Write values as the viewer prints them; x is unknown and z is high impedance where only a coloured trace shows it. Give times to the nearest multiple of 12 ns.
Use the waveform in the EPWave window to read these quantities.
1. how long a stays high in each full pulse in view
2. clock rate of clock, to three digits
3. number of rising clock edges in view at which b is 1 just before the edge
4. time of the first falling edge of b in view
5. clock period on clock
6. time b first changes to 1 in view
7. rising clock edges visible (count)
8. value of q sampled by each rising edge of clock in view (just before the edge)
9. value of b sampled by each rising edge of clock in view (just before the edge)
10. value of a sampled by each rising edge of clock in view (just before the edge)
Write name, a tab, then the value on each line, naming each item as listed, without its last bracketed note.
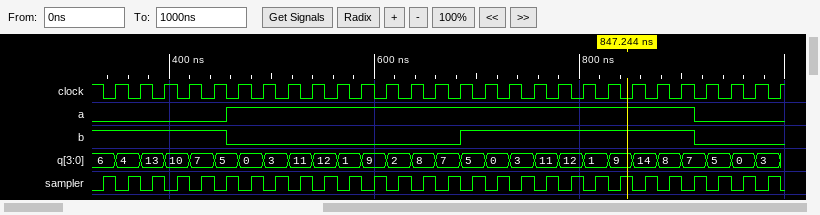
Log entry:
how long a stays high in each full pulse in view	456 ns
clock rate of clock, to three digits	41.7 MHz
number of rising clock edges in view at which b is 1 just before the edge	14
time of the first falling edge of b in view	456 ns
clock period on clock	24 ns
time b first changes to 1 in view	684 ns
rising clock edges visible	28
value of q sampled by each rising edge of clock in view	6, 4, 13, 10, 7, 5, 0, 3, 11, 12, 1, 9, 2, 8, 7, 5, 0, 3, 11, 12, 1, 9, 14, 8, 7, 5, 0, 3
value of b sampled by each rising edge of clock in view	1 1 1 1 1 0 0 0 0 0 0 0 0 0 0 1 1 1 1 1 1 1 1 1 0 0 0 0
value of a sampled by each rising edge of clock in view	0 0 0 0 0 1 1 1 1 1 1 1 1 1 1 1 1 1 1 1 1 1 1 1 0 0 0 0
